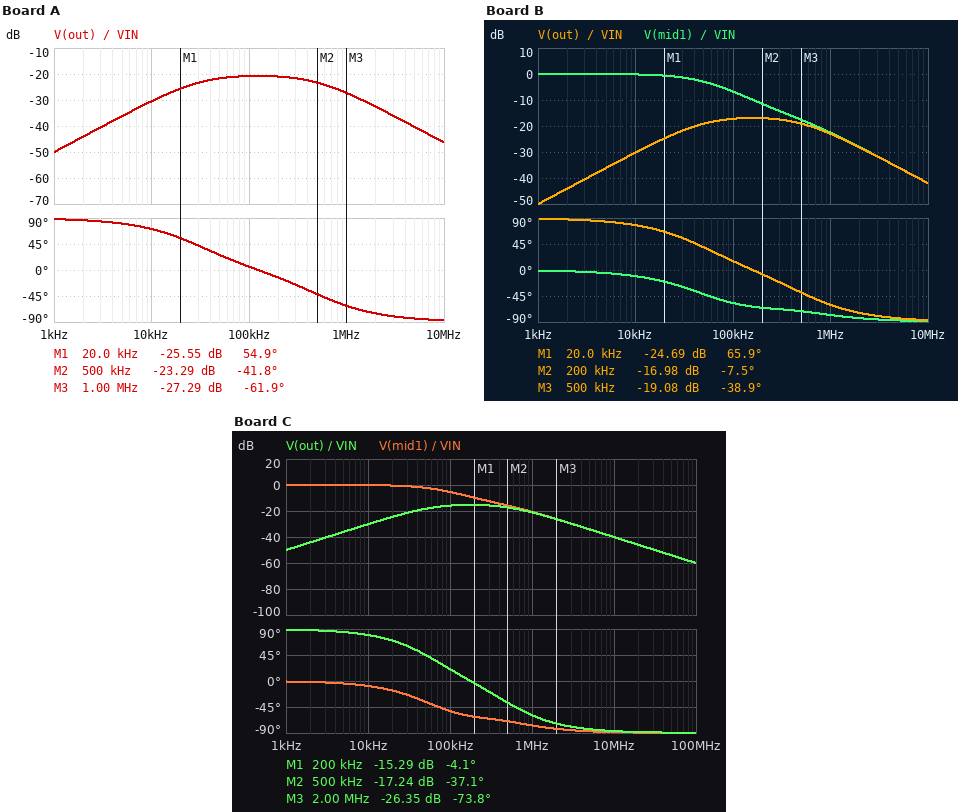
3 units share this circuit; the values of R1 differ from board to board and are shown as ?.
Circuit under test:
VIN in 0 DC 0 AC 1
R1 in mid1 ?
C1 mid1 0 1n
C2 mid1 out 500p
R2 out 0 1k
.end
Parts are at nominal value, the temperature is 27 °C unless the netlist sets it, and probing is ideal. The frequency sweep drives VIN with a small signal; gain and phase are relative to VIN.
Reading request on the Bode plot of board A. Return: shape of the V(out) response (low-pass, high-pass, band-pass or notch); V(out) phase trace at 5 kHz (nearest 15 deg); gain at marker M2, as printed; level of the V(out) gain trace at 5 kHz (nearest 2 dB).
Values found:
band-pass
75 deg
-23.29 dB
-36 dB
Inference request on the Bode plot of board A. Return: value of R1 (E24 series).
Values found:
3.3 kΩ
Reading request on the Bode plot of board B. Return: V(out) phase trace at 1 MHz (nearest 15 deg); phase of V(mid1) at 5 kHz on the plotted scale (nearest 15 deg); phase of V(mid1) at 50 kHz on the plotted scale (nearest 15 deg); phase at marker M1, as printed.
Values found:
-60 deg
0 deg
-45 deg
65.9 deg
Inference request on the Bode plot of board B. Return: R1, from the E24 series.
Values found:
2 kΩ
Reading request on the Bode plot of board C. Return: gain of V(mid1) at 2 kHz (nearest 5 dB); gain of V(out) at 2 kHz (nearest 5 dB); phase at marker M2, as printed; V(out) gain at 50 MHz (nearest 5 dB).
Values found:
0 dB
-45 dB
-37.1 deg
-55 dB
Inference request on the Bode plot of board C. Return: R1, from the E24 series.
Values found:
1.6 kΩ
